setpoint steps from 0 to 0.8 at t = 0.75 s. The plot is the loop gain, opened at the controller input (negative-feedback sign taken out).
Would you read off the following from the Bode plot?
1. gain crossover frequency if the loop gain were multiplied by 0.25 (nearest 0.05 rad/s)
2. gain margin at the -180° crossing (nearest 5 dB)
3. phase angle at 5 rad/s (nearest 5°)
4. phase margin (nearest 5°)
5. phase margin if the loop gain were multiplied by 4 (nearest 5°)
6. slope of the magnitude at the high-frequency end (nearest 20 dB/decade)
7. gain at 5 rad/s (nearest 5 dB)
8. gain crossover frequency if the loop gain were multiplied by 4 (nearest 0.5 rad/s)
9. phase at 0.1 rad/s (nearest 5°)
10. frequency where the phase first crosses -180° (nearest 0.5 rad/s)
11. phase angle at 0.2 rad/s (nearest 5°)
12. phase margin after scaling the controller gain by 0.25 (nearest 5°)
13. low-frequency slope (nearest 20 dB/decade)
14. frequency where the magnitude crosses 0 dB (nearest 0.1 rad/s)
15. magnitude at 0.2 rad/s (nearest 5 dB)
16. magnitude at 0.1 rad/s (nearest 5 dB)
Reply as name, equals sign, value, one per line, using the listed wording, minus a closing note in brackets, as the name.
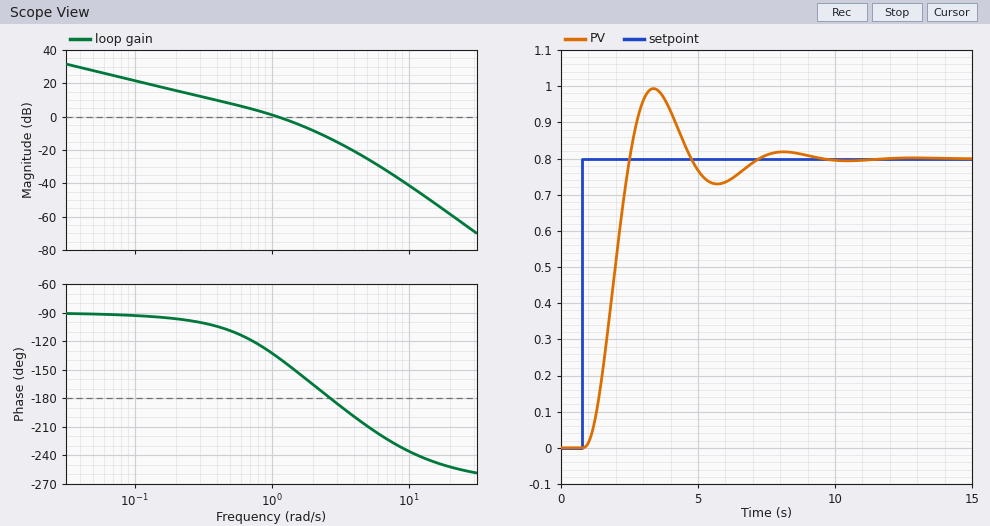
gain crossover frequency if the loop gain were multiplied by 0.25 = 0.30 rad/s
gain margin at the -180° crossing = 15 dB
phase angle at 5 rad/s = -210°
phase margin = 45°
phase margin if the loop gain were multiplied by 4 = 5°
slope of the magnitude at the high-frequency end = -60 dB/decade
gain at 5 rad/s = -25 dB
gain crossover frequency if the loop gain were multiplied by 4 = 2.5 rad/s
phase at 0.1 rad/s = -95°
frequency where the phase first crosses -180° = 2.5 rad/s
phase angle at 0.2 rad/s = -95°
phase margin after scaling the controller gain by 0.25 = 80°
low-frequency slope = -20 dB/decade
frequency where the magnitude crosses 0 dB = 1.1 rad/s
magnitude at 0.2 rad/s = 15 dB
magnitude at 0.1 rad/s = 20 dB
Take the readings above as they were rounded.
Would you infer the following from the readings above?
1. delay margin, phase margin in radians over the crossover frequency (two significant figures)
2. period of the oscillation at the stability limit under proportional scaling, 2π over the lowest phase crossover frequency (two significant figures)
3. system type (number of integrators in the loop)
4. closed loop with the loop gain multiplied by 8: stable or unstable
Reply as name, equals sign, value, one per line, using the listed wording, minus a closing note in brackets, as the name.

delay margin, phase margin in radians over the crossover frequency = 0.71 s
period of the oscillation at the stability limit under proportional scaling, 2π over the lowest phase crossover frequency = 2.5 s
system type = 1
closed loop with the loop gain multiplied by 8: stable or unstable = unstable
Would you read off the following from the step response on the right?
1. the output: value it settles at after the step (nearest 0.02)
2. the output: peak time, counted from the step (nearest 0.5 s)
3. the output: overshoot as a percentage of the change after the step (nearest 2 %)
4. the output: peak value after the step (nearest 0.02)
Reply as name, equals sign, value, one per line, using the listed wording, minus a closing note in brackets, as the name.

the output: value it settles at after the step = 0.80
the output: peak time, counted from the step = 2.5 s
the output: overshoot as a percentage of the change after the step = 24 %
the output: peak value after the step = 1.00
